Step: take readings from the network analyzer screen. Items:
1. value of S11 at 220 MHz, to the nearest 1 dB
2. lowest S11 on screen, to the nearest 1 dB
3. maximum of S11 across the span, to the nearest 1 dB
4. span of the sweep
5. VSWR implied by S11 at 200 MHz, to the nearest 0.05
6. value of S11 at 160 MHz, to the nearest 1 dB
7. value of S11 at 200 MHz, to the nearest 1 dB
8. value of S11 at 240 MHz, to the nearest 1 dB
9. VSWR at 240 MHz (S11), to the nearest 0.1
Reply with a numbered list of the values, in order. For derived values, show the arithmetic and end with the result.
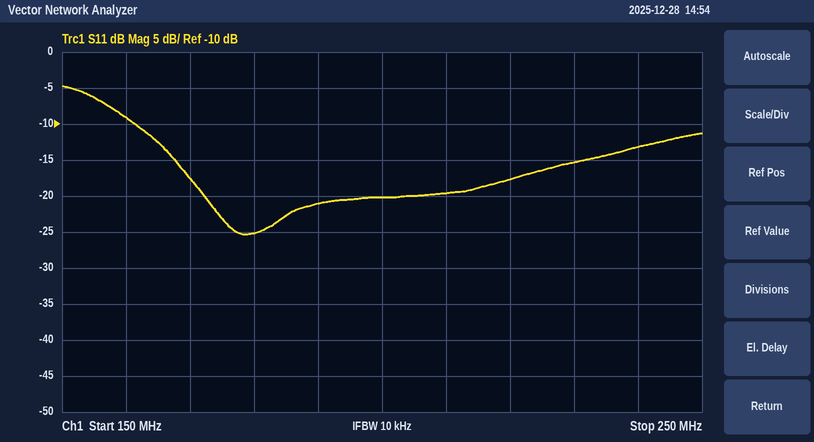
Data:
1. -18 dB
2. -25 dB
3. -5 dB
4. 100 MHz
5. |Γ| = 10^(-20/20) = 0.1000; VSWR = (1 + 0.1000)/(1 − 0.1000) ≈ 1.22, so 1.20 to the nearest 0.05
6. -9 dB
7. -20 dB
8. -13 dB
9. |Γ| = 10^(-13/20) = 0.2239; VSWR = (1 + 0.2239)/(1 − 0.2239) ≈ 1.6
